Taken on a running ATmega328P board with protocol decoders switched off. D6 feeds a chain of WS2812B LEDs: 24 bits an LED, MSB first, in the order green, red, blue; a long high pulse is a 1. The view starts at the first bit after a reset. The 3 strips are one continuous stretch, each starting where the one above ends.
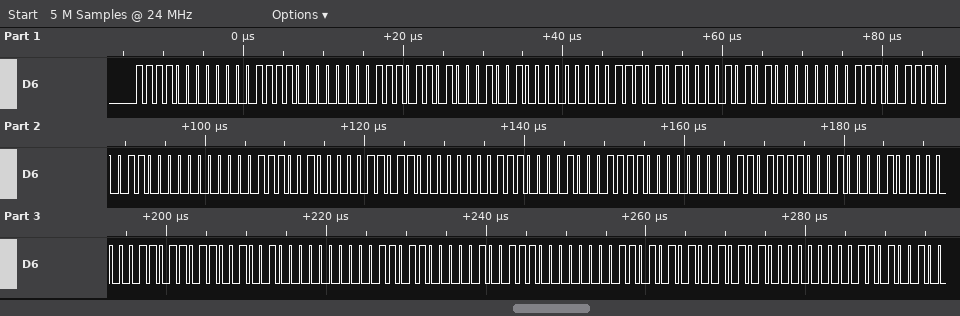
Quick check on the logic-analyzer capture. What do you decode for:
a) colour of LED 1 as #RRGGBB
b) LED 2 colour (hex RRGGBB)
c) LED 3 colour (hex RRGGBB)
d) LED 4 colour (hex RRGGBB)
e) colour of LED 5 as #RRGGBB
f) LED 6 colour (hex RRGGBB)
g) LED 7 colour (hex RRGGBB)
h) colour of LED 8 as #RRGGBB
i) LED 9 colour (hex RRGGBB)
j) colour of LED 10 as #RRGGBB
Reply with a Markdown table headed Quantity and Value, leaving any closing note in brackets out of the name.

| Quantity | Value |
|---|---|
| colour of LED 1 as #RRGGBB | #0FF000 |
| LED 2 colour | #12ED00 |
| LED 3 colour | #15EA00 |
| LED 4 colour | #18E700 |
| colour of LED 5 as #RRGGBB | #1BE400 |
| LED 6 colour | #1EE100 |
| LED 7 colour | #21DE00 |
| colour of LED 8 as #RRGGBB | #24DB00 |
| LED 9 colour | #27D800 |
| colour of LED 10 as #RRGGBB | #2AD500 |
